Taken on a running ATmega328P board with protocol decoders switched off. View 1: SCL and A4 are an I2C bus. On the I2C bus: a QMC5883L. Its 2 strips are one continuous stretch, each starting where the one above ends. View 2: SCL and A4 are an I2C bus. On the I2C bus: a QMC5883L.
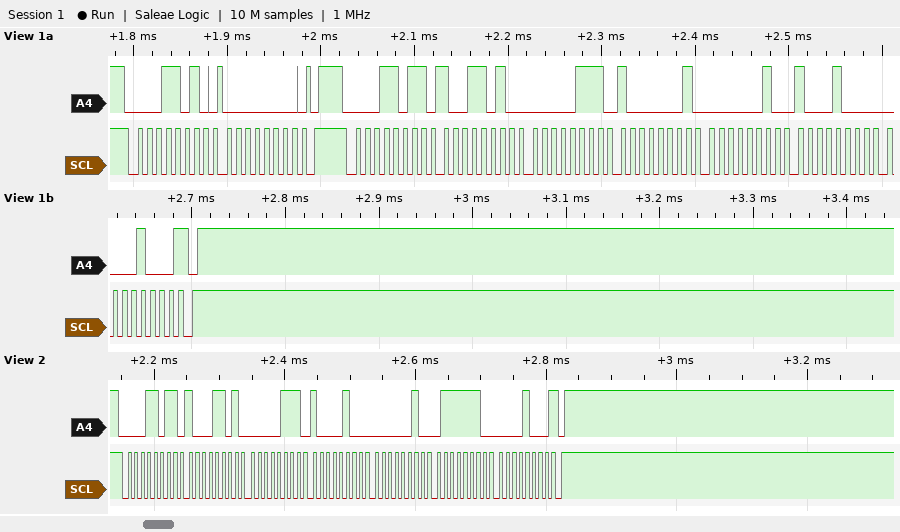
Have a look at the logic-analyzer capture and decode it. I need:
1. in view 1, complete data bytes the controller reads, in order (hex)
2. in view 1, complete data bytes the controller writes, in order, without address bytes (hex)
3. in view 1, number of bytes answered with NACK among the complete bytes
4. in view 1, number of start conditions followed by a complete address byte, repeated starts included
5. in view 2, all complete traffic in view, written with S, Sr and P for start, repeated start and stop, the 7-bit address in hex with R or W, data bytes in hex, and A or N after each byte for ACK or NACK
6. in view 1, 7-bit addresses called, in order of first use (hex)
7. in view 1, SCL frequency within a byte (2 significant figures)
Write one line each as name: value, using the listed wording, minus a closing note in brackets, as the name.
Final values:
in view 1, complete data bytes the controller reads, in order: 9A 07 81 02 88 08
in view 1, complete data bytes the controller writes, in order, without address bytes: 00
in view 1, number of bytes answered with NACK among the complete bytes: 1
in view 1, number of start conditions followed by a complete address byte, repeated starts included: 2
in view 2, all complete traffic in view, written with S, Sr and P for start, repeated start and stop, the 7-bit address in hex with R or W, data bytes in hex, and A or N after each byte for ACK or NACK: S 0DR A 8D A 07 A 84 A 02 A 7E A 08 N P
in view 1, 7-bit addresses called, in order of first use: 0x0D
in view 1, SCL frequency within a byte: 100 kHz
